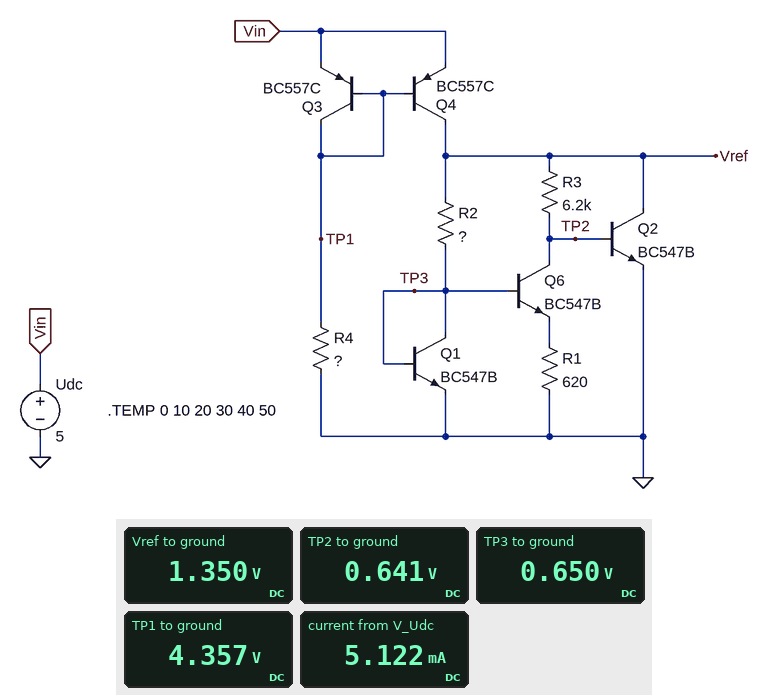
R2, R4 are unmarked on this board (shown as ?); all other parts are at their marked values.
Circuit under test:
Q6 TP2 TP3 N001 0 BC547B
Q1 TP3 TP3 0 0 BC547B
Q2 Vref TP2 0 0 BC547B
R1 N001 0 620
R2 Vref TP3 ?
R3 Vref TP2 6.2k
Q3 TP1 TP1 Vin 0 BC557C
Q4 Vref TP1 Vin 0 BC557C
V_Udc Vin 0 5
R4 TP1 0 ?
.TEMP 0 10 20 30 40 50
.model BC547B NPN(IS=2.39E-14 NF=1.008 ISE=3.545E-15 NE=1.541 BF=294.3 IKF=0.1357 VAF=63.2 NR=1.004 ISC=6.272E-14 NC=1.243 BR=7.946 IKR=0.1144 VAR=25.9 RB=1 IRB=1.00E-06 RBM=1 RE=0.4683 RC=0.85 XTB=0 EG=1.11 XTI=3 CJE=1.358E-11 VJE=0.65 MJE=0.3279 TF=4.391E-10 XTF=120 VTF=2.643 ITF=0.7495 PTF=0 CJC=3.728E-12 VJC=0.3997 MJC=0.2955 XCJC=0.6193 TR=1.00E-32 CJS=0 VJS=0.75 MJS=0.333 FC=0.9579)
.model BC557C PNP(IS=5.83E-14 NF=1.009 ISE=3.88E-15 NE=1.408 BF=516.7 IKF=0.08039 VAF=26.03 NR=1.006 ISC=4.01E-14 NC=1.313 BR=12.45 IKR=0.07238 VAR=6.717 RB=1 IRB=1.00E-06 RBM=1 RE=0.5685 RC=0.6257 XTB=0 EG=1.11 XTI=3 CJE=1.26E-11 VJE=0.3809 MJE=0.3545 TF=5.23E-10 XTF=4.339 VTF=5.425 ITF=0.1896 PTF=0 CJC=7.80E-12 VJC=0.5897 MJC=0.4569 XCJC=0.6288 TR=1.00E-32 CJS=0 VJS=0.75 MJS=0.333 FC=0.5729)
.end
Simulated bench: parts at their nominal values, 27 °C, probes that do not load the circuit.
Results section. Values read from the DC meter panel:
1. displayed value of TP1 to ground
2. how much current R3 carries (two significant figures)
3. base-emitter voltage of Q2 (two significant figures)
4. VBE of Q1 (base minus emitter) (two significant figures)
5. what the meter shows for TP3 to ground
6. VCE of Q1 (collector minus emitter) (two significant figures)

4.357 V
110 µA
640 mV
650 mV
0.650 V
650 mV
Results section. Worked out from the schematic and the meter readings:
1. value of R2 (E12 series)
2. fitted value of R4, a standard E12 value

470 Ω
1.8 kΩ
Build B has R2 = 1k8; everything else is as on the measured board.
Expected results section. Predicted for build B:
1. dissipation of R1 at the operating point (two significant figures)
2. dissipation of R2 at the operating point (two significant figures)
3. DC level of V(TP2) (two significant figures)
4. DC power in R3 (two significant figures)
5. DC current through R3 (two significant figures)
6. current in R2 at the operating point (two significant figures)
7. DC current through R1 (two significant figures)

2.4 µW
140 µW
660 mV
31 µW
71 µA
280 µA
63 µA
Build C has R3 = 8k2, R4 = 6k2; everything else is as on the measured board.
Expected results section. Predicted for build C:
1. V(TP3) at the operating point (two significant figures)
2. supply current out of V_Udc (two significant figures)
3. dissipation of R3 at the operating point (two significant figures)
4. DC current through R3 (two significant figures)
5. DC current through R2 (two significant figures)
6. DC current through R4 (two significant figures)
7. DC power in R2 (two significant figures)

630 mV
1.5 mA
64 µW
88 µA
720 µA
710 µA
240 µW
